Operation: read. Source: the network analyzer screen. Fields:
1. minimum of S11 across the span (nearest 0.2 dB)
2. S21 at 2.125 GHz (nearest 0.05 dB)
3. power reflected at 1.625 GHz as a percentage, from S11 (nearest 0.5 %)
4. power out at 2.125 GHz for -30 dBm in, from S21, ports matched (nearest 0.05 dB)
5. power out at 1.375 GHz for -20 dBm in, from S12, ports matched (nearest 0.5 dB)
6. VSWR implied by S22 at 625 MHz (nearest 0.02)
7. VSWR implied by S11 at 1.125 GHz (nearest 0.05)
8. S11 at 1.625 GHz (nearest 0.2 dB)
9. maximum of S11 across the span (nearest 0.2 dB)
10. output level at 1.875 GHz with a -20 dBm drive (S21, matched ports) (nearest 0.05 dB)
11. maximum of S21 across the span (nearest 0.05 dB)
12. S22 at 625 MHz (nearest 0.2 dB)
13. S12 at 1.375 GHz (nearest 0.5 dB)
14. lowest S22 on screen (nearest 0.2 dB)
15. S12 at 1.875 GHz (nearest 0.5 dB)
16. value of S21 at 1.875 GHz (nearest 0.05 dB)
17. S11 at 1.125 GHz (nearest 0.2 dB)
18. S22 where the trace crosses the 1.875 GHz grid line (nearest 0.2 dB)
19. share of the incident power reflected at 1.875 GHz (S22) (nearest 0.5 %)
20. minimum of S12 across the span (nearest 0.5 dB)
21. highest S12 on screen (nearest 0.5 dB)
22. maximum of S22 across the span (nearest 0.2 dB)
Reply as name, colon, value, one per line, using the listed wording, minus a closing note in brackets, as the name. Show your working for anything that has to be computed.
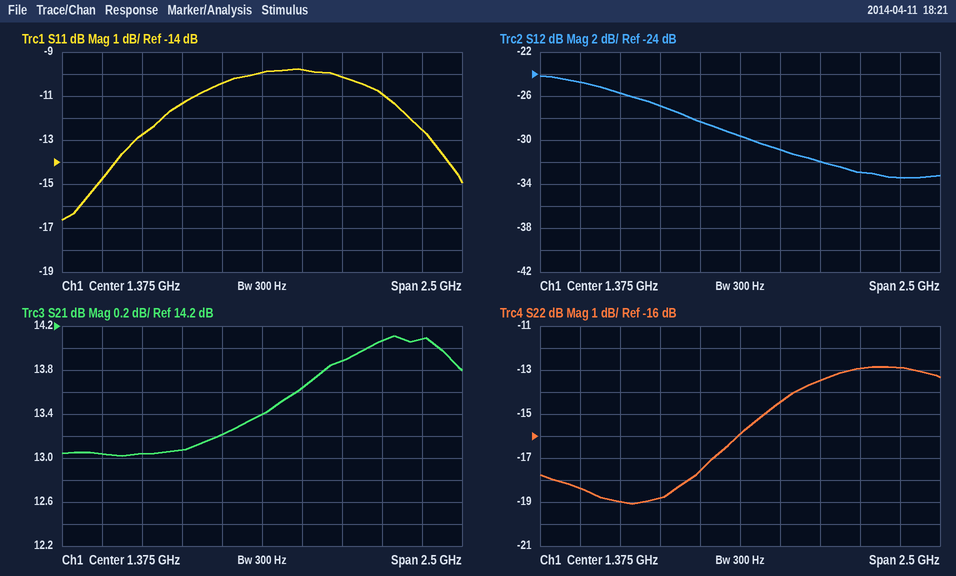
minimum of S11 across the span: -16.6 dB
S21 at 2.125 GHz: 14.05 dB
power reflected at 1.625 GHz as a percentage, from S11: 10^(-9.8/10) ≈ 10.5 %
power out at 2.125 GHz for -30 dBm in, from S21, ports matched: -30 dBm + (14.05 dB) = -15.95 dBm
power out at 1.375 GHz for -20 dBm in, from S12, ports matched: -20 dBm + (-29.5 dB) = -49.5 dBm
VSWR implied by S22 at 625 MHz: |Γ| = 10^(-19/20) = 0.1122; VSWR = (1 + 0.1122)/(1 − 0.1122) ≈ 1.25, so 1.26 to the nearest 0.02
VSWR implied by S11 at 1.125 GHz: |Γ| = 10^(-10.4/20) = 0.3020; VSWR = (1 + 0.3020)/(1 − 0.3020) ≈ 1.87, so 1.85 to the nearest 0.05
S11 at 1.625 GHz: -9.8 dB
maximum of S11 across the span: -9.8 dB
output level at 1.875 GHz with a -20 dBm drive (S21, matched ports): -20 dBm + (13.90 dB) = -6.10 dBm
maximum of S21 across the span: 14.10 dB
S22 at 625 MHz: -19.0 dB
S12 at 1.375 GHz: -29.5 dB
lowest S22 on screen: -19.0 dB
S12 at 1.875 GHz: -32.0 dB
value of S21 at 1.875 GHz: 13.90 dB
S11 at 1.125 GHz: -10.4 dB
S22 where the trace crosses the 1.875 GHz grid line: -13.4 dB
share of the incident power reflected at 1.875 GHz (S22): 10^(-13.4/10) ≈ 4.57 %, so 4.5 % to the nearest 0.5 %
minimum of S12 across the span: -33.5 dB
highest S12 on screen: -24.0 dB
maximum of S22 across the span: -12.8 dB
